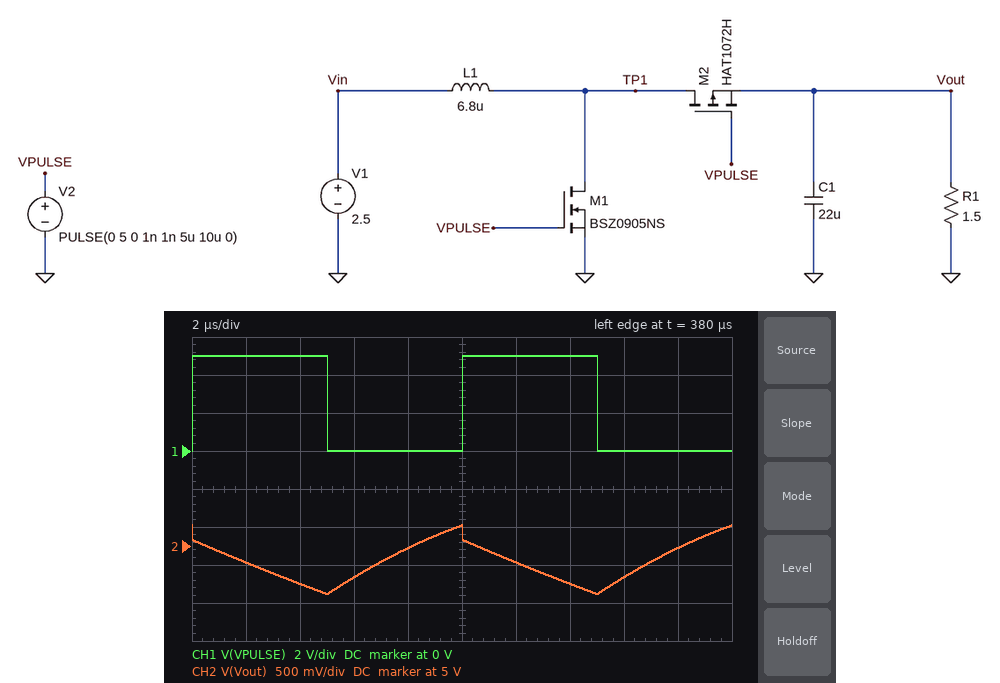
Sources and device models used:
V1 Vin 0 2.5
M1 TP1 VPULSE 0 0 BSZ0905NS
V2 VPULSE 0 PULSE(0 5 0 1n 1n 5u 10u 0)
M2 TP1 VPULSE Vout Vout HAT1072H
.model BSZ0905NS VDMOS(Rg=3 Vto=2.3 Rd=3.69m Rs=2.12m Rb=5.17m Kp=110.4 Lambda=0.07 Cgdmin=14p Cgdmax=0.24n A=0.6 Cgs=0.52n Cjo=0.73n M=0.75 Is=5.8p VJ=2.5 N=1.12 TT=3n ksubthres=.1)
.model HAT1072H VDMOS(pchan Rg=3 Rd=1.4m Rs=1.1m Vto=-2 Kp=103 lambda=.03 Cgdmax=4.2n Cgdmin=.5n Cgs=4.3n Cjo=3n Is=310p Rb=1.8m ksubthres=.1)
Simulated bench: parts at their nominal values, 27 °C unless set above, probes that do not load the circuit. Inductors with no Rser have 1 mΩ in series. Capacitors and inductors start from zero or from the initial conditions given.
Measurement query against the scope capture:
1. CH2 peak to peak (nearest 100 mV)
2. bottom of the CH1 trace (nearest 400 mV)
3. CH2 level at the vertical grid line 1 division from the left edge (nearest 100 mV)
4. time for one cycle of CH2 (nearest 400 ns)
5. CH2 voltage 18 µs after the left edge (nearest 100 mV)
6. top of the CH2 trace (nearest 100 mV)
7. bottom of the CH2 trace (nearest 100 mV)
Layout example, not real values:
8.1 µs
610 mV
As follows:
900 mV
0 V
4.8 V
10.0 µs
5.0 V
5.3 V
4.4 V
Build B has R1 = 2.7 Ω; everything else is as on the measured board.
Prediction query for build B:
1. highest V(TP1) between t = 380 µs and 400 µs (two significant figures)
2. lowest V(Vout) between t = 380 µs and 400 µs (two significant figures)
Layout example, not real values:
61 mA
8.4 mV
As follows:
5.2 V
4.6 V
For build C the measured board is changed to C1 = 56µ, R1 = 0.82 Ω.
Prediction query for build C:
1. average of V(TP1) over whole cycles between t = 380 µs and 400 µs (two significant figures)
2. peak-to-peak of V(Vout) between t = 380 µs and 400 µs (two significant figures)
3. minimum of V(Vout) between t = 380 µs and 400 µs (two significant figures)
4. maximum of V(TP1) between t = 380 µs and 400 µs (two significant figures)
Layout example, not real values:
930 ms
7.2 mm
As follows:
2.5 V
590 mV
4.5 V
5.1 V
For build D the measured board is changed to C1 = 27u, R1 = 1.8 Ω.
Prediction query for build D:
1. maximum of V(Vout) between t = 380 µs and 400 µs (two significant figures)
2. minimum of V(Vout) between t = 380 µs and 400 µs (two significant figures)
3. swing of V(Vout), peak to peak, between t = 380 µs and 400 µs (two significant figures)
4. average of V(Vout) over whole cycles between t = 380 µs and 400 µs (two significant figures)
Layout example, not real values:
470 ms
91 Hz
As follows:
5.2 V
4.5 V
640 mV
4.8 V
